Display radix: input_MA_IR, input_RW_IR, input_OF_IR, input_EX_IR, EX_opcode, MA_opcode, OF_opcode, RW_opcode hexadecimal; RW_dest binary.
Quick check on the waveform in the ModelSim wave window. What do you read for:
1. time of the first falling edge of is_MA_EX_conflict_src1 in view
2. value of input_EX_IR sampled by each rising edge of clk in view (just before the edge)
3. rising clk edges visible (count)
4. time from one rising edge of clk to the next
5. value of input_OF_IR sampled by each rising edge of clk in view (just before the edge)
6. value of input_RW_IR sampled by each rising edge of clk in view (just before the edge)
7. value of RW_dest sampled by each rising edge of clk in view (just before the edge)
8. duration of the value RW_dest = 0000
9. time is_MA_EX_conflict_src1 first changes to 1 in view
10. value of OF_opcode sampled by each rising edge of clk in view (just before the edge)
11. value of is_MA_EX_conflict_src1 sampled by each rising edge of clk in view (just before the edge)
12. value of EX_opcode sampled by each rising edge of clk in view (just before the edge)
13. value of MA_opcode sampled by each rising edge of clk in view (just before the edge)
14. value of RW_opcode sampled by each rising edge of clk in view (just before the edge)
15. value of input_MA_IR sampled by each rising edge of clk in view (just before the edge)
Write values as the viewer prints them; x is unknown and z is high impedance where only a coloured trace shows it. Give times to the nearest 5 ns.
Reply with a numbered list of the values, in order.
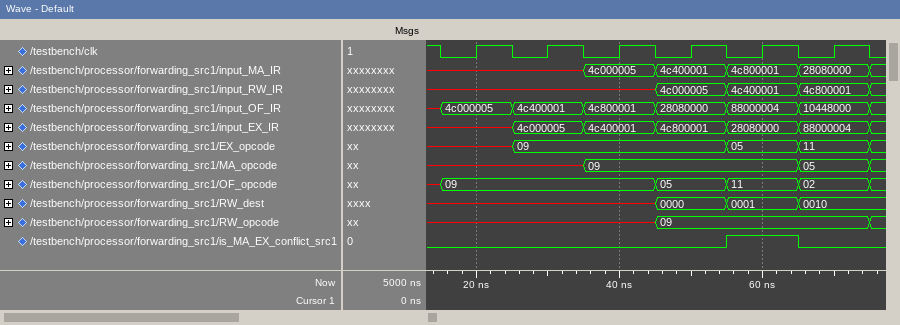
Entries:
1. 65 ns
2. x, 4c000005, 4c400001, 4c800001, 28080000, 88000004
3. 6
4. 10 ns
5. 4c000005, 4c400001, 4c800001, 28080000, 88000004, 10448000
6. x, x, x, 4c000005, 4c400001, 4c800001
7. x, x, x, 0000, 0001, 0010
8. 10 ns
9. 55 ns
10. 09, 09, 09, 05, 11, 02
11. 0 0 0 0 1 0
12. x, 09, 09, 09, 05, 11
13. x, x, 09, 09, 09, 05
14. x, x, x, 09, 09, 09
15. x, x, 4c000005, 4c400001, 4c800001, 28080000
